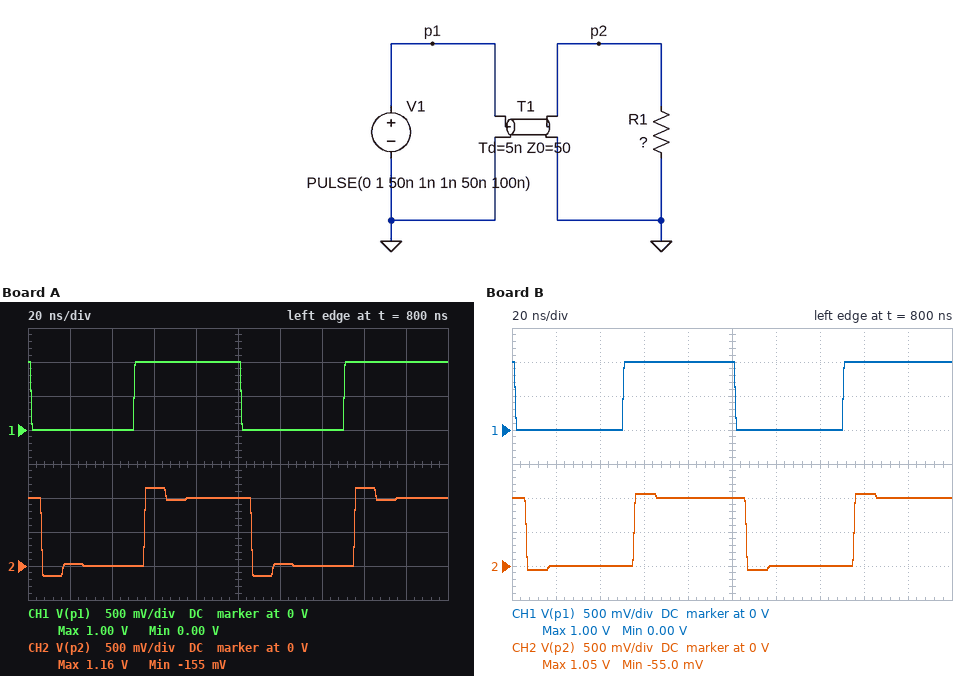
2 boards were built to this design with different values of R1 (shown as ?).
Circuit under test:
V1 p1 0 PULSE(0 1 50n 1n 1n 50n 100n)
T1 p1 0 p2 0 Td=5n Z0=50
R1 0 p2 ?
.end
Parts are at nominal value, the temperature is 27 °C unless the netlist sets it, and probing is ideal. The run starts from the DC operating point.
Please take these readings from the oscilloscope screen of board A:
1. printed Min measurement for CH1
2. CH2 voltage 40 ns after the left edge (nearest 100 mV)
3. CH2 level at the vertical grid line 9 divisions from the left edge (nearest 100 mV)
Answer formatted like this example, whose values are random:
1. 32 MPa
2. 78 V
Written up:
1. 0.00 V
2. 0 V
3. 1.0 V
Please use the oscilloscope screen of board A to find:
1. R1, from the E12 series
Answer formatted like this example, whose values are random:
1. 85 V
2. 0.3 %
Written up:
1. 68 Ω
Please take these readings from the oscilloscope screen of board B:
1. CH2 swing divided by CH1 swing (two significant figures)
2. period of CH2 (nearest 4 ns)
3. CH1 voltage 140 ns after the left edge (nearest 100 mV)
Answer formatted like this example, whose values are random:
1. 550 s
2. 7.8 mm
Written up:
1. 1.1
2. 100 ns
3. 0 V
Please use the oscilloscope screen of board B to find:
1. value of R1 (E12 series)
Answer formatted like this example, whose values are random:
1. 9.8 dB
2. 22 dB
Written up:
1. 56 Ω
